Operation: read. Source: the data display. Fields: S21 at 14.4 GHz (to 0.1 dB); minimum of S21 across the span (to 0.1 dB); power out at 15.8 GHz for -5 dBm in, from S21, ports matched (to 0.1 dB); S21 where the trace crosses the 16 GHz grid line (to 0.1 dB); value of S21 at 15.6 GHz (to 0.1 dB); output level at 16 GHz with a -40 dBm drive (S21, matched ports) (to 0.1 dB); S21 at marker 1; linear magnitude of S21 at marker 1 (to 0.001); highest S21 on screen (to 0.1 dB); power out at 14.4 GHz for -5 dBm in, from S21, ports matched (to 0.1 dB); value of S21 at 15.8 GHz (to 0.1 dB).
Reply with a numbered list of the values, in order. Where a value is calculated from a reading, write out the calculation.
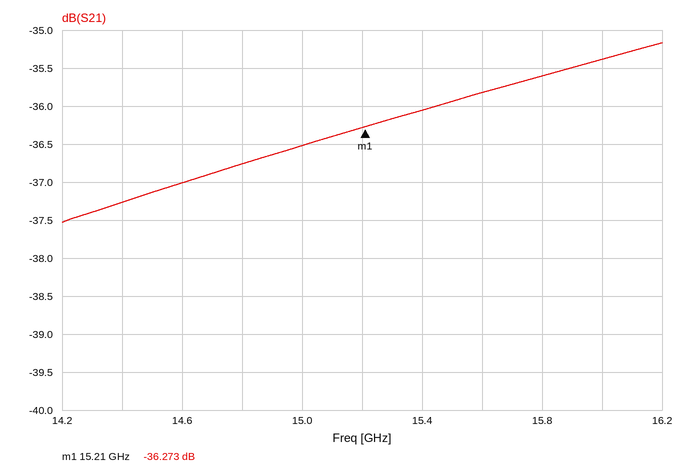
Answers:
1. -37.3 dB
2. -37.5 dB
3. -5 dBm + (-35.6 dB) = -40.6 dBm
4. -35.4 dB
5. -35.8 dB
6. -40 dBm + (-35.4 dB) = -75.4 dBm
7. -36.273 dB
8. 10^(-36.273/20) ≈ 0.015
9. -35.2 dB
10. -5 dBm + (-37.3 dB) = -42.3 dBm
11. -35.6 dB
